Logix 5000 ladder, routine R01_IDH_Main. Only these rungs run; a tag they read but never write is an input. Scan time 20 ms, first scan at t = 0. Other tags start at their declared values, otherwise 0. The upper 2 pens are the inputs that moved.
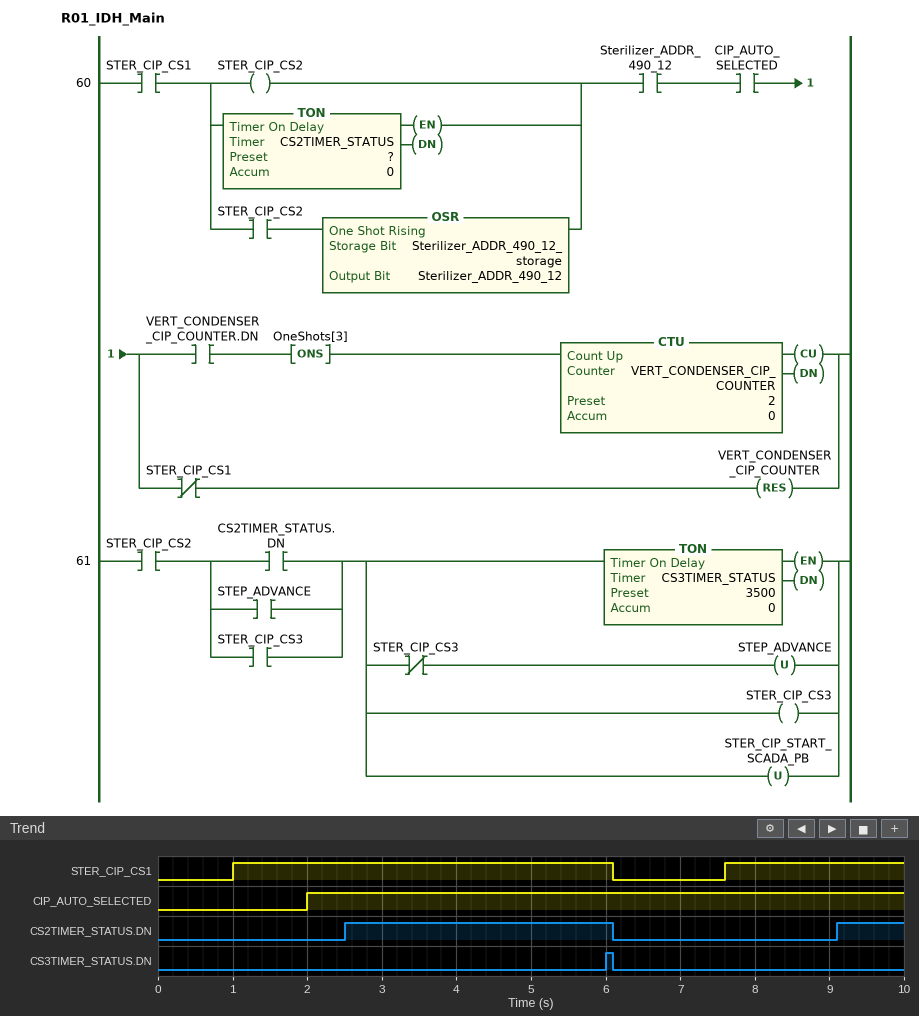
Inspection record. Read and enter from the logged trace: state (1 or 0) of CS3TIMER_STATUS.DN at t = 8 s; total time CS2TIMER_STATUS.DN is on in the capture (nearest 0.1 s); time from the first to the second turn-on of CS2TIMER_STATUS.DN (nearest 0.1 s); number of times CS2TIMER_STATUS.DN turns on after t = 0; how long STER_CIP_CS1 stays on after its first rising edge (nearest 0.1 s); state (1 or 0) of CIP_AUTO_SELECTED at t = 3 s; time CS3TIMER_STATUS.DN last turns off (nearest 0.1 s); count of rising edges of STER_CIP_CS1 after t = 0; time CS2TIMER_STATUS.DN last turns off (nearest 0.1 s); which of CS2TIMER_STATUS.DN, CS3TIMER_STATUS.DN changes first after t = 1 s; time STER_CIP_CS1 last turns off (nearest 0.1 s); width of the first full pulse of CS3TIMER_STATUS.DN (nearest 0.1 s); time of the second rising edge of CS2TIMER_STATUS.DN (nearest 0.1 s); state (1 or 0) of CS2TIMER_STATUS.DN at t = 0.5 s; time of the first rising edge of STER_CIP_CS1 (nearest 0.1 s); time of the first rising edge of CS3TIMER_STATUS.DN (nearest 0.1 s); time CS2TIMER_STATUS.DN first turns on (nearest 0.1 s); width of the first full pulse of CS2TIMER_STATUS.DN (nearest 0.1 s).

0
4.5 s
6.6 s
2
5.1 s
1
6.1 s
2
6.1 s
CS2TIMER_STATUS.DN
6.1 s
0.1 s
9.1 s
0
1.0 s
6.0 s
2.5 s
3.6 s
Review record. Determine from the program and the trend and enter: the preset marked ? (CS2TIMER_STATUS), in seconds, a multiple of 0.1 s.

1.5 s
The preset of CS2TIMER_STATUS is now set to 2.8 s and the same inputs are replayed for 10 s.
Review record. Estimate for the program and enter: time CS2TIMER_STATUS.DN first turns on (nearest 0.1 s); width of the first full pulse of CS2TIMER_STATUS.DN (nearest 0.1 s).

3.8 s
2.3 s
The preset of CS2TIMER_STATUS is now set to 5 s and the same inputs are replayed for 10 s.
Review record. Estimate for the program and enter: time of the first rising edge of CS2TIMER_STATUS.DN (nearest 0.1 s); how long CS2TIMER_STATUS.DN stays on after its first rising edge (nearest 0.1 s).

6.0 s
0.1 s
